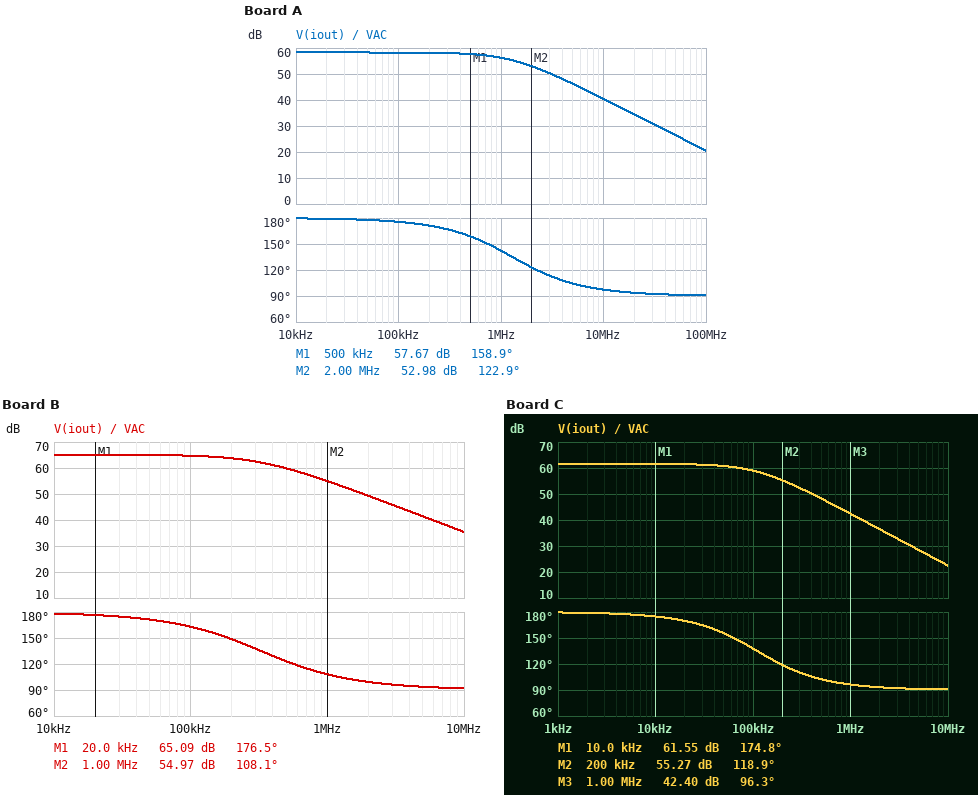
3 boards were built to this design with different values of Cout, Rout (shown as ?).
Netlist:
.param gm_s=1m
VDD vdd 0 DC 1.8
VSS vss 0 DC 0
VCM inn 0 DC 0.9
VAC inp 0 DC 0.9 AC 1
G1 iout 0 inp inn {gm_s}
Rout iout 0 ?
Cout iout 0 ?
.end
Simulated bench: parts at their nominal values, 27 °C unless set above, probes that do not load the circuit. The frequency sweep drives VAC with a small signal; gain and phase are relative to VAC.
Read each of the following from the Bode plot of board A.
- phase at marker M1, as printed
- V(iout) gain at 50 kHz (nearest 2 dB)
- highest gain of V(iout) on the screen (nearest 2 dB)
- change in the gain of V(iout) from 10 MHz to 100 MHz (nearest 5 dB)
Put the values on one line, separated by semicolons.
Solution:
158.9 deg; 58 dB; 58 dB; -20 dB
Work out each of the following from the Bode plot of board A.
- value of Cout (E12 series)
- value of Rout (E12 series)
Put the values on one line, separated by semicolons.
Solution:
150 fF; 820 kΩ
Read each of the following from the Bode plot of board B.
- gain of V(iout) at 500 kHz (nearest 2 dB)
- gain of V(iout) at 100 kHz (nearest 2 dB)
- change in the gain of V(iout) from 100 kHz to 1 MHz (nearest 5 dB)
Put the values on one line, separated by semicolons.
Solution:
60 dB; 64 dB; -10 dB
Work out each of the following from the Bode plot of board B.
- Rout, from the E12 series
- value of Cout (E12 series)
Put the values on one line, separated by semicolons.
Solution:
1.8 MΩ; 270 fF
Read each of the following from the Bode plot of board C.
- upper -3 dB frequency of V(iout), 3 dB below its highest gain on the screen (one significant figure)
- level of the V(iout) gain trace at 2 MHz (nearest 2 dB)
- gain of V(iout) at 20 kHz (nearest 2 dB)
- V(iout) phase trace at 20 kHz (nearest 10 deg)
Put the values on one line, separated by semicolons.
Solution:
100 kHz; 36 dB; 62 dB; 170 deg
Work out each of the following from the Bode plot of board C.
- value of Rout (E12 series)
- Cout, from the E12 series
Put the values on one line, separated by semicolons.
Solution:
1.2 MΩ; 1.2 pF
